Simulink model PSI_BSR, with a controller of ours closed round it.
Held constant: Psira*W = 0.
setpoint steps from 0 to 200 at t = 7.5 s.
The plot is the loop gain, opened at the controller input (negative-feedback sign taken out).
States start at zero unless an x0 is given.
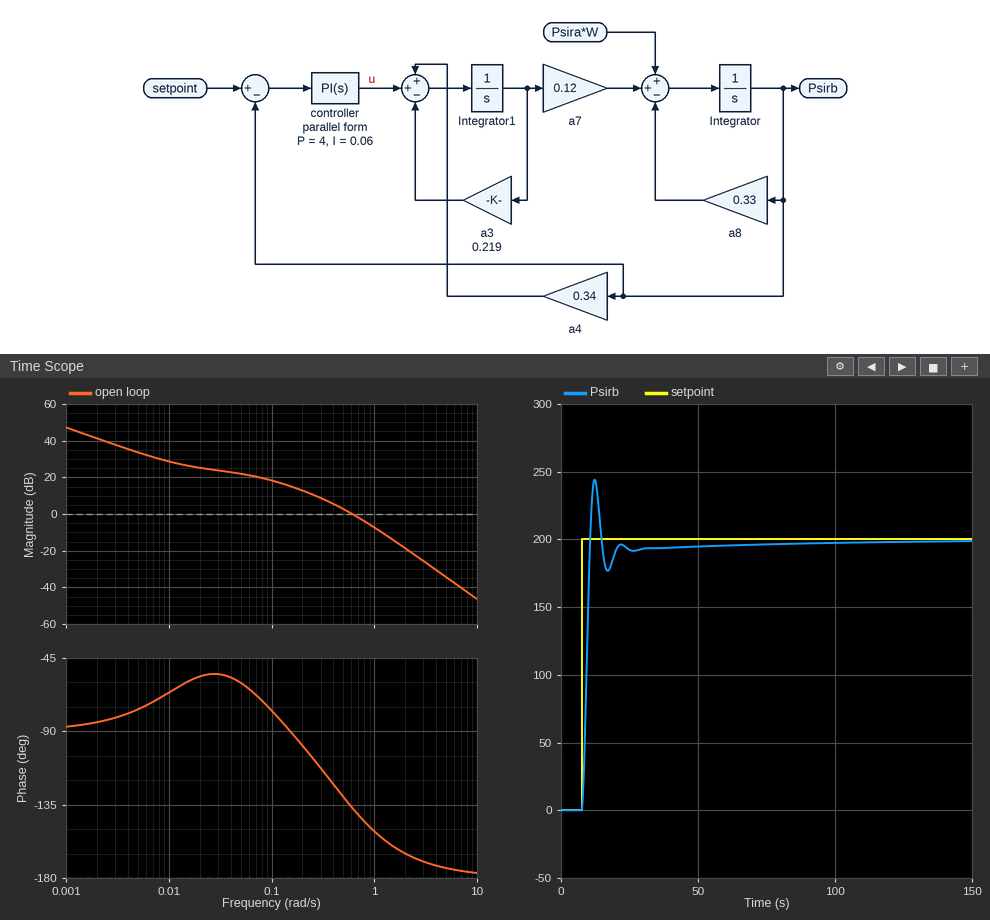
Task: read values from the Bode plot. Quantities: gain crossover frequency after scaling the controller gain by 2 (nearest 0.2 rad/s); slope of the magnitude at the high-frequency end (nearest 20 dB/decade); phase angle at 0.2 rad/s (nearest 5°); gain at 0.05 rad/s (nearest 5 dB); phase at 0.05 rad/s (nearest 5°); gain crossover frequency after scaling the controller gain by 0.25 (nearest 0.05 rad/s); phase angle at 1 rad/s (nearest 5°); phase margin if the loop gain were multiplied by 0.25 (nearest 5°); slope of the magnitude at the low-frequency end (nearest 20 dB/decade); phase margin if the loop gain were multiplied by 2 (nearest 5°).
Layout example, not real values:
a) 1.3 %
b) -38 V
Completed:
a) 1.0 rad/s
b) -40 dB/decade
c) -100°
d) 20 dB
e) -60°
f) 0.20 rad/s
g) -150°
h) 80°
i) -20 dB/decade
j) 30°
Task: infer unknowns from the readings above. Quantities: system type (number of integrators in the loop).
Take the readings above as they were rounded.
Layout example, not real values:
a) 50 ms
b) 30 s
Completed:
a) 1
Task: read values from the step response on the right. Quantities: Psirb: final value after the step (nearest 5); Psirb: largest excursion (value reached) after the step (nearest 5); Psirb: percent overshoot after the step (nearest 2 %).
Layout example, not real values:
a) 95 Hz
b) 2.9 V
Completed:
a) 200
b) 245
c) 22 %
